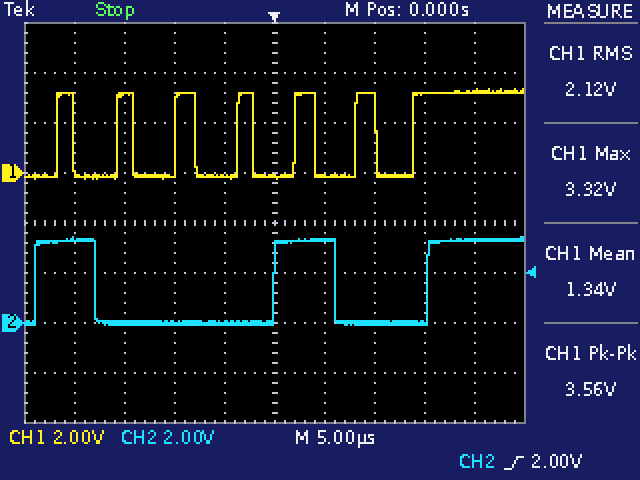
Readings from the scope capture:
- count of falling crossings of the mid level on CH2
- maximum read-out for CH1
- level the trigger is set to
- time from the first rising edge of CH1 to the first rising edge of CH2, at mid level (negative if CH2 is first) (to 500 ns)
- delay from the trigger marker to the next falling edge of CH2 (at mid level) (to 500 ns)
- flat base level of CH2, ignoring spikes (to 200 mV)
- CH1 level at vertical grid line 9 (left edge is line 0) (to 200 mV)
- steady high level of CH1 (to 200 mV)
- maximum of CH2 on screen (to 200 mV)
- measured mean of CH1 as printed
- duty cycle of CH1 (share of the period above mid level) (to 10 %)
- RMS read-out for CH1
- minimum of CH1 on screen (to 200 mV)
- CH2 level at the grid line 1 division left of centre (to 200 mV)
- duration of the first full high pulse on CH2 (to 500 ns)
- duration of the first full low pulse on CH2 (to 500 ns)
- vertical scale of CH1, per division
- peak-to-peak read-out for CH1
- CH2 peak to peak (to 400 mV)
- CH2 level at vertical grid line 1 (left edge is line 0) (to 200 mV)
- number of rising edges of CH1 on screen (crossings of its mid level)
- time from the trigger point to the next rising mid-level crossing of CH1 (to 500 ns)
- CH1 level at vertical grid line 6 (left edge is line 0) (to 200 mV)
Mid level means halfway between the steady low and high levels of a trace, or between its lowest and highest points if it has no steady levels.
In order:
2
3.32 V
2.00 V
-2.0 µs
6.0 µs
0.0 V
3.2 V
3.2 V
3.4 V
1.34 V
30 %
2.12 V
-200 mV
0.0 V
6.0 µs
18.0 µs
2 V
3.56 V
3.6 V
3.4 V
7
2.0 µs
-200 mV
